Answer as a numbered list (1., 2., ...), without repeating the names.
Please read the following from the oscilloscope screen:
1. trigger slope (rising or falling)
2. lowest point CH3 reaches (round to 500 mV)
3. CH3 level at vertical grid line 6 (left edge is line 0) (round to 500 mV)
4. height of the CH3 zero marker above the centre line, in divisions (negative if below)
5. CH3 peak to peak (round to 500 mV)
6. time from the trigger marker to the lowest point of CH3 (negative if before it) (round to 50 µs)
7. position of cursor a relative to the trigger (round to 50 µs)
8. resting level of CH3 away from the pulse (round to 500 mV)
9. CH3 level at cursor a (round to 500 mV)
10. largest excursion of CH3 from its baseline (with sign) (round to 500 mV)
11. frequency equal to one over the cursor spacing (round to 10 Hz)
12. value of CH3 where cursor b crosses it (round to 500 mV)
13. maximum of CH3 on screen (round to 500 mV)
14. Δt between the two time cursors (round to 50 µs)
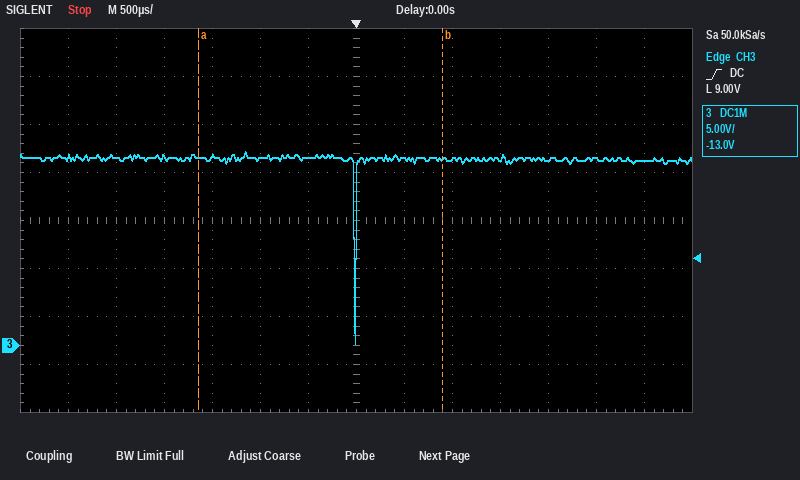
1. rising
2. 0.0 V
3. 19.5 V
4. -2.6 div
5. 20.0 V
6. 0 µs
7. -1.65 ms
8. 19.5 V
9. 19.5 V
10. -19.5 V
11. 390 Hz
12. 19.5 V
13. 20.0 V
14. 2.55 ms
